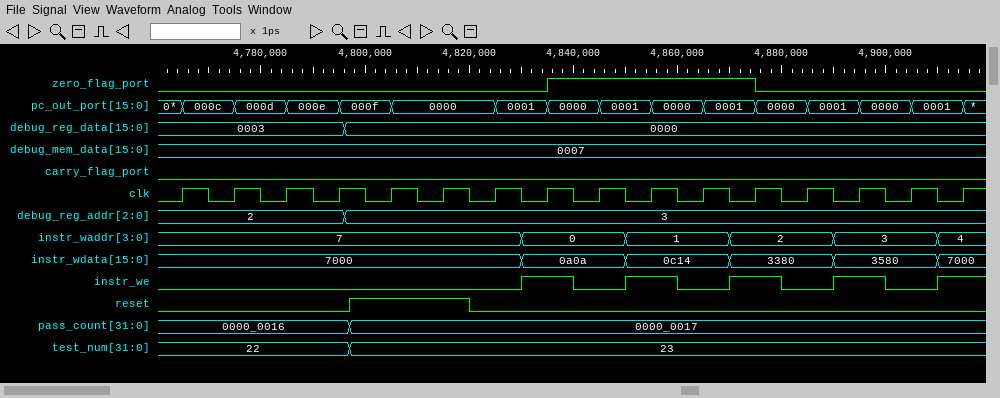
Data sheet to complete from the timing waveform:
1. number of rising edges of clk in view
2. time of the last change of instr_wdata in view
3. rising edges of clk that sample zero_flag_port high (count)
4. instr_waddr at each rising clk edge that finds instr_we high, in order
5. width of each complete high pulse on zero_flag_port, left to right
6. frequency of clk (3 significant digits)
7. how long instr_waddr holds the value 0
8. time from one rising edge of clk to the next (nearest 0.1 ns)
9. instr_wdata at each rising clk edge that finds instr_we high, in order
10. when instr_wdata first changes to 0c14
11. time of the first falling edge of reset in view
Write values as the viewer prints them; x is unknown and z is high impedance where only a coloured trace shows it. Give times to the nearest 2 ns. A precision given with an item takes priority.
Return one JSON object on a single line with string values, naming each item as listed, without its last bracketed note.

{"number of rising edges of clk in view": "16", "time of the last change of instr_wdata in view": "4910 ns", "rising edges of clk that sample zero_flag_port high": "4", "instr_waddr at each rising clk edge that finds instr_we high, in order": "0, 1, 2, 3, 4", "width of each complete high pulse on zero_flag_port, left to right": "40 ns", "frequency of clk": "100 MHz", "how long instr_waddr holds the value 0": "20 ns", "time from one rising edge of clk to the next": "10 ns", "instr_wdata at each rising clk edge that finds instr_we high, in order": "0a0a, 0c14, 3380, 3580, 7000", "when instr_wdata first changes to 0c14": "4850 ns", "time of the first falling edge of reset in view": "4820 ns"}
